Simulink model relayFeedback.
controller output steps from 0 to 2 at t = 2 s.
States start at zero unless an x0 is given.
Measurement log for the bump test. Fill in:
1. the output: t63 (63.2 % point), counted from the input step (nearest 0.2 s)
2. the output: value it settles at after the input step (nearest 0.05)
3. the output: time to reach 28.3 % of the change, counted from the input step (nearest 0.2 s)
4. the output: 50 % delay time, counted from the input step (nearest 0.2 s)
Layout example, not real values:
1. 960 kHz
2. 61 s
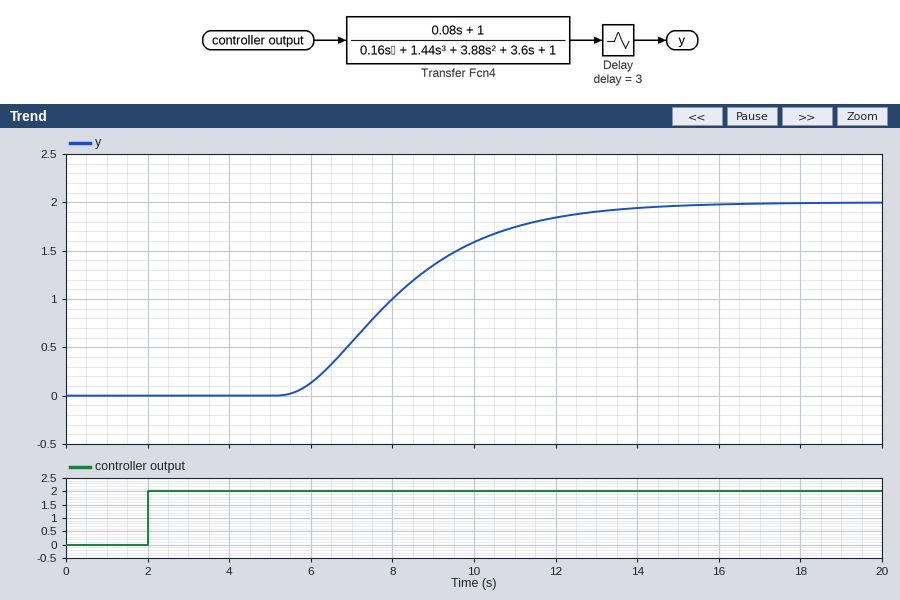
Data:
1. 6.8 s
2. 2.00
3. 5.0 s
4. 6.0 s
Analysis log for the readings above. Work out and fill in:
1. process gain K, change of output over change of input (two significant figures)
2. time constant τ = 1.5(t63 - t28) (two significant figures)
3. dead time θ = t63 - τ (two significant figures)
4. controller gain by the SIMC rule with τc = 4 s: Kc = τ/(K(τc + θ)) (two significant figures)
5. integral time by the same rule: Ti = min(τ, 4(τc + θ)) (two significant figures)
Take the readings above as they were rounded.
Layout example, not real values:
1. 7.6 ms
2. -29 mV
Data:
1. 1.0
2. 2.7 s
3. 4.1 s
4. 0.33
5. 2.7 s
